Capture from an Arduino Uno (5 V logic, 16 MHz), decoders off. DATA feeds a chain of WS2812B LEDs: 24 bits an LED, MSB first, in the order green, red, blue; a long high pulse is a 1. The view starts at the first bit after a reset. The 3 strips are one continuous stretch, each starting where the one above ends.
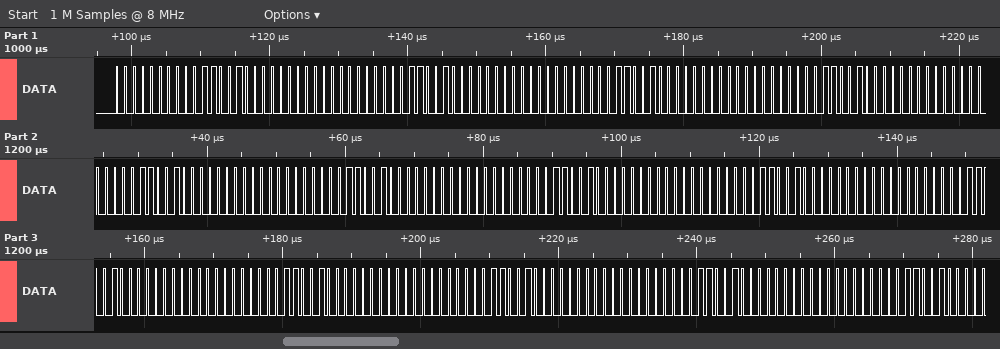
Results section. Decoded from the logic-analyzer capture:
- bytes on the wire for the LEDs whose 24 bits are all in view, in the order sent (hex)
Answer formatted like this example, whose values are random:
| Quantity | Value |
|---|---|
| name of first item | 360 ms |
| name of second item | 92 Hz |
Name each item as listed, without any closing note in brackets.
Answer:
| Quantity | Value |
|---|---|
| bytes on the wire for the LEDs whose 24 bits are all in view, in the order sent | 00 32 00 00 32 00 00 32 00 00 32 00 00 32 00 00 32 00 00 32 00 00 32 00 00 32 00 00 32 00 00 32 00 00 32 00 |
